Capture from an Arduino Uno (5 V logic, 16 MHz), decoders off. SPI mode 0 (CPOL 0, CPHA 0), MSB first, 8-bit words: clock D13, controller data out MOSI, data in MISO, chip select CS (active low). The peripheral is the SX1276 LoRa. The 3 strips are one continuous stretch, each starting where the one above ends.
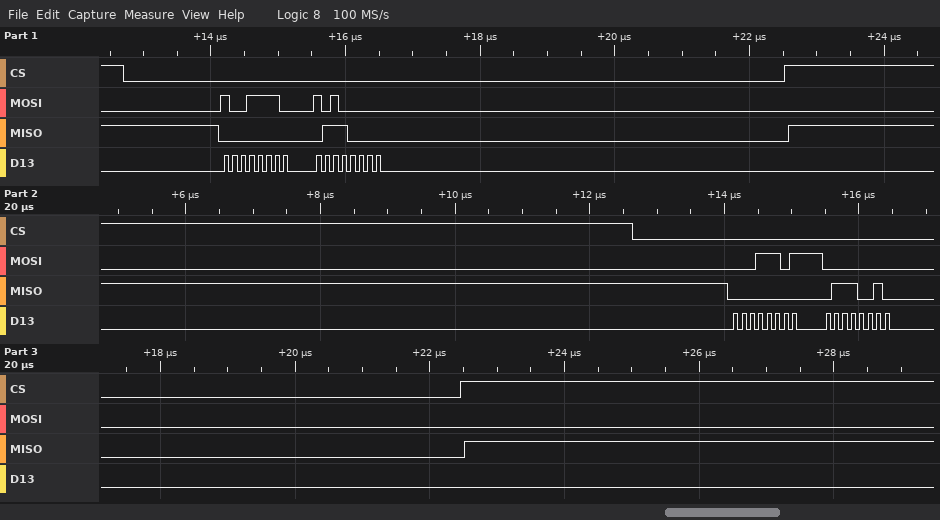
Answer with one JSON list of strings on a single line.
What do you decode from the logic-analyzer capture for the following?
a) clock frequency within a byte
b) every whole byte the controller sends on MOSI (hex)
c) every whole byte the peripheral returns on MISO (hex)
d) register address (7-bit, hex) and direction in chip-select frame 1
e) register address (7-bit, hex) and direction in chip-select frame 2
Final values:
["8 MHz", "9E A0 1D 00", "00 70 00 72", "0x1E write", "0x1D read"]
